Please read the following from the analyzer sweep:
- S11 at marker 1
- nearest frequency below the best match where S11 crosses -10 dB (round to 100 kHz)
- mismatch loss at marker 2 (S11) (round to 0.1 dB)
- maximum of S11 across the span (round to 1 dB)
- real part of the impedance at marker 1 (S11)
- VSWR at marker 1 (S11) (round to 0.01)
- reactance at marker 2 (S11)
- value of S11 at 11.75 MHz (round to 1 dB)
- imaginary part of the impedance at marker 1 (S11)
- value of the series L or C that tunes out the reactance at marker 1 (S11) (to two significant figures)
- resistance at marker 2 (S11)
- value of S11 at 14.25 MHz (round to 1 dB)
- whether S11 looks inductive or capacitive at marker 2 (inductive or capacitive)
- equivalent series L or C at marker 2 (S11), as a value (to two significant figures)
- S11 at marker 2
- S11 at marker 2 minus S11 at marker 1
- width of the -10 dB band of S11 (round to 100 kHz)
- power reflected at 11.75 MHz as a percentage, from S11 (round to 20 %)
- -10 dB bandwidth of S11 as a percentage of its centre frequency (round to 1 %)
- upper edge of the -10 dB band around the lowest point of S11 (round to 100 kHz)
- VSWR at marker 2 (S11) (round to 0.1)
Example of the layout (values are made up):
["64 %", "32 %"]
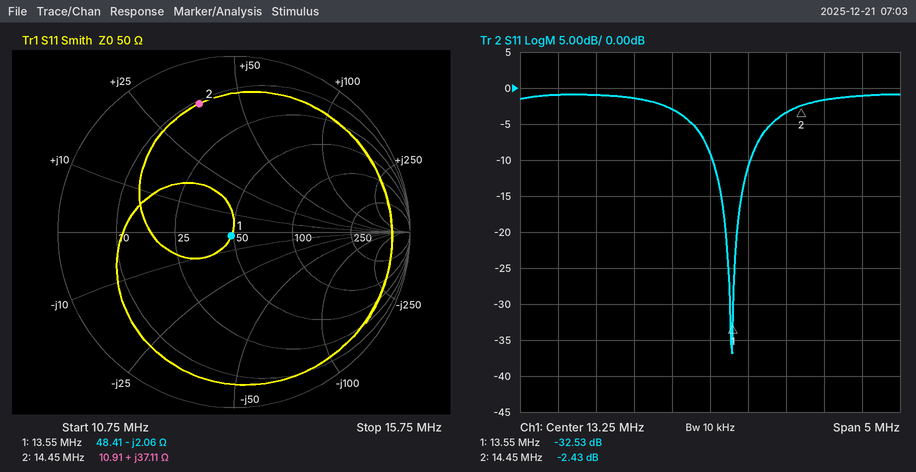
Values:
["-32.53 dB", "13.3 MHz", "3.7 dB", "-1 dB", "48.41 Ω", "1.05", "+37.11 Ω", "-1 dB", "-2.06 Ω", "24 nH", "10.91 Ω", "-3 dB", "inductive", "410 nH", "-2.43 dB", "30.10 dB", "500 kHz", "80 %", "4 %", "13.8 MHz", "7.2"]
